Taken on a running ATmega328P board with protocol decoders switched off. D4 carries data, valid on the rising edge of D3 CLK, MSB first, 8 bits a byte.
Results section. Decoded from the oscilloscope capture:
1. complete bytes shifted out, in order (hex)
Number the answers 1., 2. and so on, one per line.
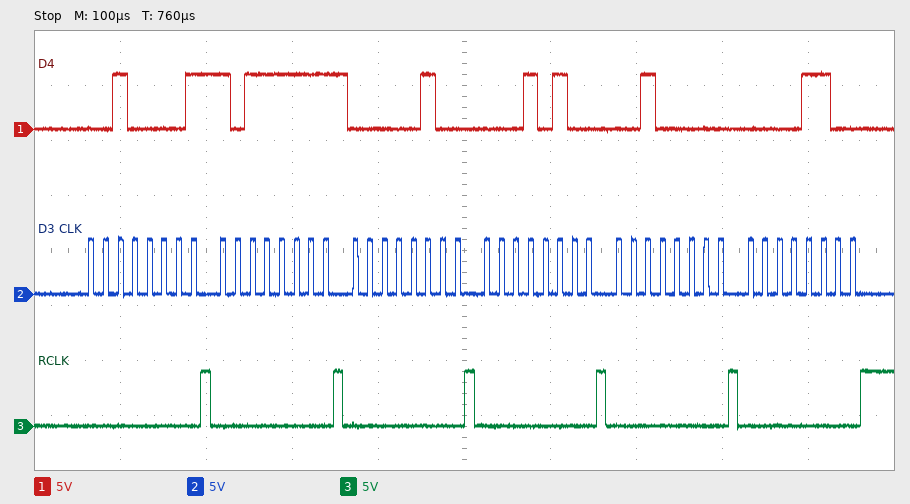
1. 21 BF 04 14 20 0C
